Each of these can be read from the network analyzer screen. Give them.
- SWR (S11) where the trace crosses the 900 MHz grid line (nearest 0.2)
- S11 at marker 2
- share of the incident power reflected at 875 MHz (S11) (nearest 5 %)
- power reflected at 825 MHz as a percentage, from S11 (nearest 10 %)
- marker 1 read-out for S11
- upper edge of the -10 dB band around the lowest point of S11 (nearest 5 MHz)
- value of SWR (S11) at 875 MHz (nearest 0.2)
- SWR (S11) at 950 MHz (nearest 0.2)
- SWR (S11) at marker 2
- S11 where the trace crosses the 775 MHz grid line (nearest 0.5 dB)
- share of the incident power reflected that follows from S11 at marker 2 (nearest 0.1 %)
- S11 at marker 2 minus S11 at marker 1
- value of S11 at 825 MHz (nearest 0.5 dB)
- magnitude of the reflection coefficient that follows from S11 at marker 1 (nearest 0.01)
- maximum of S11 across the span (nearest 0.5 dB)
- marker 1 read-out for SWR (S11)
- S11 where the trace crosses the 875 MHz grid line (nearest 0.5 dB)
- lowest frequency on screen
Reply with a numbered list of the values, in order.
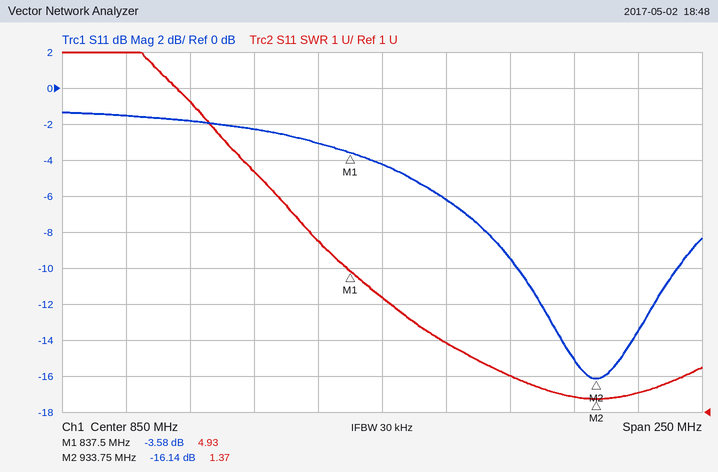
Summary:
1. 2.0
2. -16.14 dB
3. 25 %
4. 50 %
5. -3.58 dB
6. 965 MHz
7. 3.0
8. 1.6
9. 1.37
10. -2.0 dB
11. 2.4 %
12. -12.56 dB
13. -3.0 dB
14. 0.66
15. -1.5 dB
16. 4.93
17. -6.0 dB
18. 725 MHz
